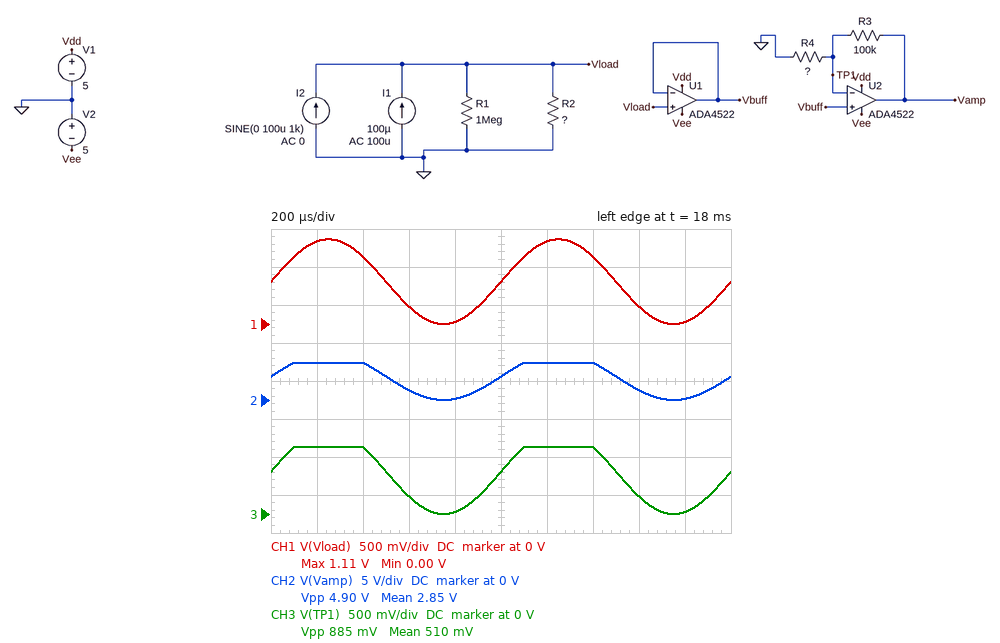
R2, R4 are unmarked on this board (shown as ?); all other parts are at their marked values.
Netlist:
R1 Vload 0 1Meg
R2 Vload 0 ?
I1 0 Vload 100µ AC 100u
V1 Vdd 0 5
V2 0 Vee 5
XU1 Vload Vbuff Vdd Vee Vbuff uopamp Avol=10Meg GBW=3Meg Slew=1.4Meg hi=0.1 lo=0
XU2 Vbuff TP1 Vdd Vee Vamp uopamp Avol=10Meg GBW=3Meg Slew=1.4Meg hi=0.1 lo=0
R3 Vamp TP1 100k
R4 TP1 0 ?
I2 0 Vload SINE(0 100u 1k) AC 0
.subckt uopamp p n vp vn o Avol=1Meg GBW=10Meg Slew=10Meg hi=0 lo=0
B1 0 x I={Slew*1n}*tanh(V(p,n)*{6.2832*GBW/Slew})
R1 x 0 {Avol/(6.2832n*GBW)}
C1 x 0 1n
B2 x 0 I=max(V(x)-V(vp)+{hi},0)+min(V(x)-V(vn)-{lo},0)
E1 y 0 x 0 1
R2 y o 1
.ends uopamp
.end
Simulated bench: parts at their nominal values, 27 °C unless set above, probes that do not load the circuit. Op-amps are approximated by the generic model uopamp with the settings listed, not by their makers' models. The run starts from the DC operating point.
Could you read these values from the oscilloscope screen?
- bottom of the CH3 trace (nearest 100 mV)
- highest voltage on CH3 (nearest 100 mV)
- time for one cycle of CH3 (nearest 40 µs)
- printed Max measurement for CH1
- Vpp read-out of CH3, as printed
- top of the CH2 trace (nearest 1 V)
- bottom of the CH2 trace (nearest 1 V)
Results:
0 V
900 mV
1.00 ms
1.11 V
885 mV
5 V
0 V
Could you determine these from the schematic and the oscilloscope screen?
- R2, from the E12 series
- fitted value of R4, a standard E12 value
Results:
5.6 kΩ
22 kΩ
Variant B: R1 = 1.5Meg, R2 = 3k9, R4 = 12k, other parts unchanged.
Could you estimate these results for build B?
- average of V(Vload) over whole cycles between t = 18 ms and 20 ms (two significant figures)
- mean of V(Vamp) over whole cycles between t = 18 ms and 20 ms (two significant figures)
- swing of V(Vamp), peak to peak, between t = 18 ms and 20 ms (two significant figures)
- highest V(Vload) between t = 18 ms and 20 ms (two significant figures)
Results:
390 mV
3.0 V
4.9 V
780 mV
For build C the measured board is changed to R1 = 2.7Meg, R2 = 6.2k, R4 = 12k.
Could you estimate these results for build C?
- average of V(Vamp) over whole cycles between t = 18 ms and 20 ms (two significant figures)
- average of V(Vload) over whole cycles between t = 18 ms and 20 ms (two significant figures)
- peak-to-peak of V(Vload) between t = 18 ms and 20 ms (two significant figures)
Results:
3.5 V
620 mV
1.2 V
